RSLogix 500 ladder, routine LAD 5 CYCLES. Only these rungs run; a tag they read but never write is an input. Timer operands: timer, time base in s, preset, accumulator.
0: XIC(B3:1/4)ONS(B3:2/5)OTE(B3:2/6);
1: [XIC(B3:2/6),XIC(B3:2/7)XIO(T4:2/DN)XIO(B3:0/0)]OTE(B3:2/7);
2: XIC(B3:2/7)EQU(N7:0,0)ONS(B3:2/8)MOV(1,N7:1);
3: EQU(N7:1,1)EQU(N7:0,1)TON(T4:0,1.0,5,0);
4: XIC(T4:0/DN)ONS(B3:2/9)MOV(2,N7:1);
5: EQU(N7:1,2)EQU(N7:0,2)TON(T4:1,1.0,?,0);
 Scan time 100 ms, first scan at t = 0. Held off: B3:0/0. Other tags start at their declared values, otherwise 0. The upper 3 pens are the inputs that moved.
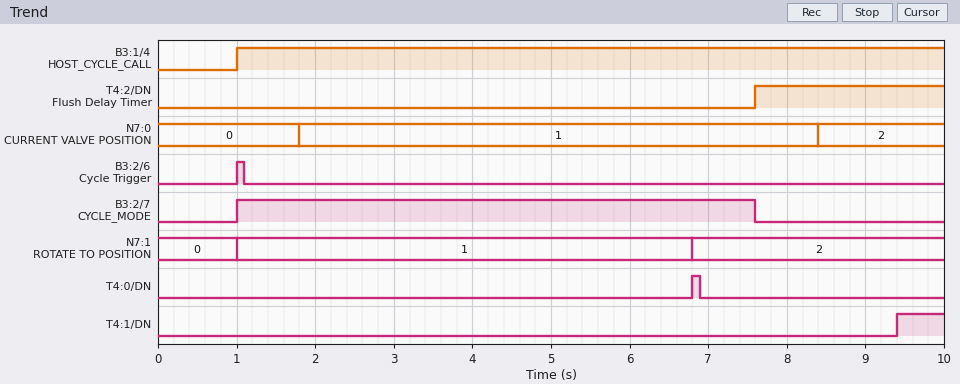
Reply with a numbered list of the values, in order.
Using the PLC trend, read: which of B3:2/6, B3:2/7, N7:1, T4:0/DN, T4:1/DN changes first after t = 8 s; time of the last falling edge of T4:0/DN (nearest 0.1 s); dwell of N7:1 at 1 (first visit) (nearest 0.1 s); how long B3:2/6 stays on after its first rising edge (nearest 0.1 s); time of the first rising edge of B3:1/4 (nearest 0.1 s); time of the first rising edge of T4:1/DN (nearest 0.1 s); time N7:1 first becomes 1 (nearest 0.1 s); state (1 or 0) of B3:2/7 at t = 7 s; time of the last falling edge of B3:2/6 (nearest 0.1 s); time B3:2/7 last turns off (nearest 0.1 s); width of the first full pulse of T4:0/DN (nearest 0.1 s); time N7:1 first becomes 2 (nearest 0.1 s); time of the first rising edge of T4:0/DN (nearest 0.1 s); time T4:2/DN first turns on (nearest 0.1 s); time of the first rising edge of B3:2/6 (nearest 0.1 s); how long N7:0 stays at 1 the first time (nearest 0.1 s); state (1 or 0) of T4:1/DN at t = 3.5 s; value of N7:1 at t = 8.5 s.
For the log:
1. T4:1/DN
2. 6.9 s
3. 5.8 s
4. 0.1 s
5. 1.0 s
6. 9.4 s
7. 1.0 s
8. 1
9. 1.1 s
10. 7.6 s
11. 0.1 s
12. 6.8 s
13. 6.8 s
14. 7.6 s
15. 1.0 s
16. 6.6 s
17. 0
18. 2
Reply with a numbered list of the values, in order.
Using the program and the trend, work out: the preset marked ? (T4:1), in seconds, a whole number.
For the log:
1. 1 s
